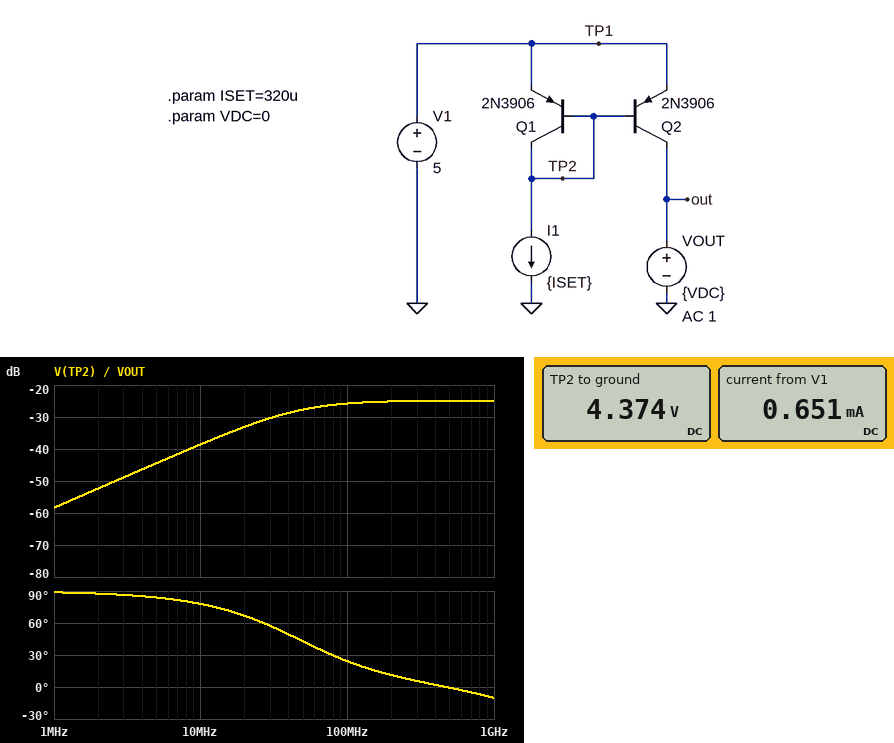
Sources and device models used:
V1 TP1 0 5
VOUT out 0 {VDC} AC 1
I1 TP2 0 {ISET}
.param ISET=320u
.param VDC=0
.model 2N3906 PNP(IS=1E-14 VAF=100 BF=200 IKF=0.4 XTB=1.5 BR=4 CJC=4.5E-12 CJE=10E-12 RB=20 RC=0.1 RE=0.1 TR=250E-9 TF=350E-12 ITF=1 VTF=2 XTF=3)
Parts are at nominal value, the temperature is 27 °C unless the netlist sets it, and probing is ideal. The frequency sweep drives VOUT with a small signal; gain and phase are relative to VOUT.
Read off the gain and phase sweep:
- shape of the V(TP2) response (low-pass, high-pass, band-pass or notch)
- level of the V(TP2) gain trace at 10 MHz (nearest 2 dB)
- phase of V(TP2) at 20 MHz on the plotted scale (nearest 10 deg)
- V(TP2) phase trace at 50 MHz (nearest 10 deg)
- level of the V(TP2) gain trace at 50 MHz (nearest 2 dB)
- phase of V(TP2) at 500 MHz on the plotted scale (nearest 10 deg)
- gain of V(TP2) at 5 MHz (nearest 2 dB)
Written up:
high-pass
-38 dB
70 deg
40 deg
-28 dB
0 deg
-44 dB
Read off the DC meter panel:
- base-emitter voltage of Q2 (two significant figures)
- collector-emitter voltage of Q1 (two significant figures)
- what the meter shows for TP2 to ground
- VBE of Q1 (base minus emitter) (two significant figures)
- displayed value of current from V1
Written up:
-630 mV
-630 mV
4.374 V
-630 mV
0.651 mA
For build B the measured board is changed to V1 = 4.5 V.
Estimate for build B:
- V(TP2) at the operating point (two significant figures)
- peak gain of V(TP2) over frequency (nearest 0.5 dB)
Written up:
3.9 V
-24.5 dB
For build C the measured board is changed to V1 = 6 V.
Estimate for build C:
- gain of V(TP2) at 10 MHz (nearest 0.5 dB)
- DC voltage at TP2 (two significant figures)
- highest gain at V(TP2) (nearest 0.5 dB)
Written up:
-39.0 dB
5.4 V
-25.5 dB
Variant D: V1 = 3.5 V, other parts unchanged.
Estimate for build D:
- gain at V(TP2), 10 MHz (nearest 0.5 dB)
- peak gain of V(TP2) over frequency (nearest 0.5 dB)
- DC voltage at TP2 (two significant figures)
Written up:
-37.5 dB
-24.0 dB
2.9 V
